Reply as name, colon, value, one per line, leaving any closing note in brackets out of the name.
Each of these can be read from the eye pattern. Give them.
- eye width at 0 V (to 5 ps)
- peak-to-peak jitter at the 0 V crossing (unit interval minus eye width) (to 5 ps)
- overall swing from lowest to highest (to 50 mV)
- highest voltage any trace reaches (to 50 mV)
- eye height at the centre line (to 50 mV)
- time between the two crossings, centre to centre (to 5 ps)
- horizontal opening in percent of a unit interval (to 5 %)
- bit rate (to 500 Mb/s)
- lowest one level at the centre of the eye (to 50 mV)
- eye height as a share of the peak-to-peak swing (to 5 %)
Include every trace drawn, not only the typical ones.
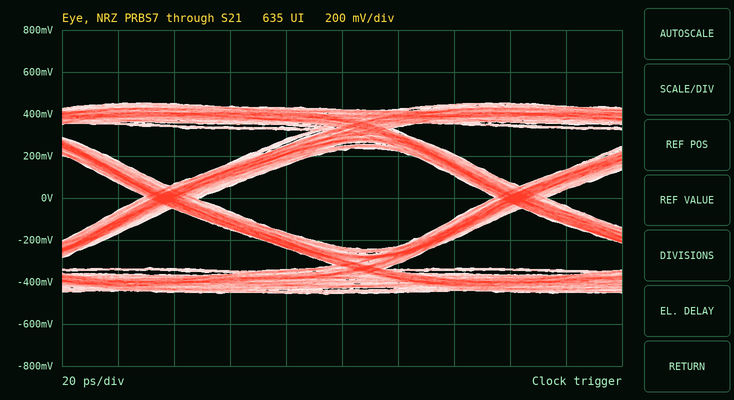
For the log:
eye width at 0 V: 105 ps
peak-to-peak jitter at the 0 V crossing (unit interval minus eye width): 20 ps
overall swing from lowest to highest: 900 mV
highest voltage any trace reaches: 450 mV
eye height at the centre line: 450 mV
time between the two crossings, centre to centre: 125 ps
horizontal opening in percent of a unit interval: 85 %
bit rate: 8.0 Gb/s
lowest one level at the centre of the eye: 250 mV
eye height as a share of the peak-to-peak swing: 50 %
